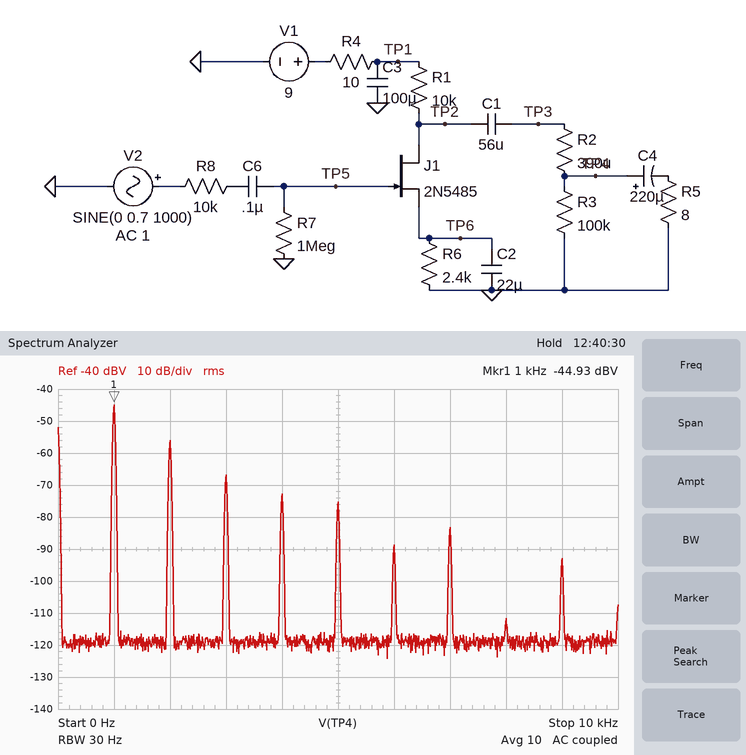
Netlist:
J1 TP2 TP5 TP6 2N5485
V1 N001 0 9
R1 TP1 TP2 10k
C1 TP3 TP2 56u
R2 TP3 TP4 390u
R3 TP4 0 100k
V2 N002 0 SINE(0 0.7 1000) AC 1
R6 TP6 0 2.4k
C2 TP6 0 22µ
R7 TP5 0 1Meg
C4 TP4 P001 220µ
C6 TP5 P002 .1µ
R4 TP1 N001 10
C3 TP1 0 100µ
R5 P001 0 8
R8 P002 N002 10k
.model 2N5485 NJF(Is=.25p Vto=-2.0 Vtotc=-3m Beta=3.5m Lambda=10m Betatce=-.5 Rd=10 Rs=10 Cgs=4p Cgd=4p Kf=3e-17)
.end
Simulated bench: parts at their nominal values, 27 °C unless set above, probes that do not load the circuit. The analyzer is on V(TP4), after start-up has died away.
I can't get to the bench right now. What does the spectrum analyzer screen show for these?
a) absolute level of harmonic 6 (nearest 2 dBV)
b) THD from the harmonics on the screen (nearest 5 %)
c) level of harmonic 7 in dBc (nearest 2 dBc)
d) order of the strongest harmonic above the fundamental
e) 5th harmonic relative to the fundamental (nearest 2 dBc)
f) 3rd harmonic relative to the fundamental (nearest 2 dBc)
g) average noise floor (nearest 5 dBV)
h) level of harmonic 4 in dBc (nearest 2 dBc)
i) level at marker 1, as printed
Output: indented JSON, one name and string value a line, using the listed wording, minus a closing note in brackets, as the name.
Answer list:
{
  "absolute level of harmonic 6": "-88 dBV",
  "THD from the harmonics on the screen": "30 %",
  "level of harmonic 7 in dBc": "-38 dBc",
  "order of the strongest harmonic above the fundamental": "2",
  "5th harmonic relative to the fundamental": "-30 dBc",
  "3rd harmonic relative to the fundamental": "-22 dBc",
  "average noise floor": "-120 dBV",
  "level of harmonic 4 in dBc": "-28 dBc",
  "level at marker 1, as printed": "-44.93 dBV"
}
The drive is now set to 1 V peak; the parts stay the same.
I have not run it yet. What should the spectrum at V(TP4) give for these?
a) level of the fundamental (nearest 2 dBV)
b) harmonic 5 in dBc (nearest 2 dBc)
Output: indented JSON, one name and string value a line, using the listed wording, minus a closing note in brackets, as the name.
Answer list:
{
  "level of the fundamental": "-44 dBV",
  "harmonic 5 in dBc": "-28 dBc"
}
